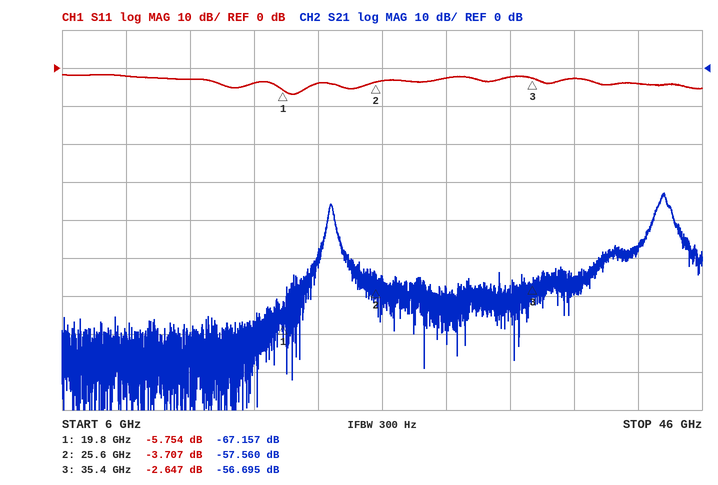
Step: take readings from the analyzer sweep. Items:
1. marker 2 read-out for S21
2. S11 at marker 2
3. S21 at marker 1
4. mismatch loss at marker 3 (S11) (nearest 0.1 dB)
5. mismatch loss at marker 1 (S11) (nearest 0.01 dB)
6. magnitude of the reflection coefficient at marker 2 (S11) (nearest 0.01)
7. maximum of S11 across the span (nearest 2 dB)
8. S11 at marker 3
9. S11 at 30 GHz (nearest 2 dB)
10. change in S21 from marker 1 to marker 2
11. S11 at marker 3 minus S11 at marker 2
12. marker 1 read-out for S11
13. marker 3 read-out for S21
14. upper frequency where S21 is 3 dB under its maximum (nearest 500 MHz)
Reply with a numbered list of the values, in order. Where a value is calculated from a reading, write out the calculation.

1. -57.560 dB
2. -3.707 dB
3. -67.157 dB
4. −10 log10(1 − 10^(-2.647/10)) ≈ 3.4 dB
5. −10 log10(1 − 10^(-5.754/10)) ≈ 1.34 dB
6. 10^(-3.707/20) ≈ 0.65
7. -2 dB
8. -2.647 dB
9. -2 dB
10. -57.56 − (-67.157) = 9.597 dB
11. -2.647 − (-3.707) = 1.060 dB
12. -5.754 dB
13. -56.695 dB
14. 44.0 GHz
